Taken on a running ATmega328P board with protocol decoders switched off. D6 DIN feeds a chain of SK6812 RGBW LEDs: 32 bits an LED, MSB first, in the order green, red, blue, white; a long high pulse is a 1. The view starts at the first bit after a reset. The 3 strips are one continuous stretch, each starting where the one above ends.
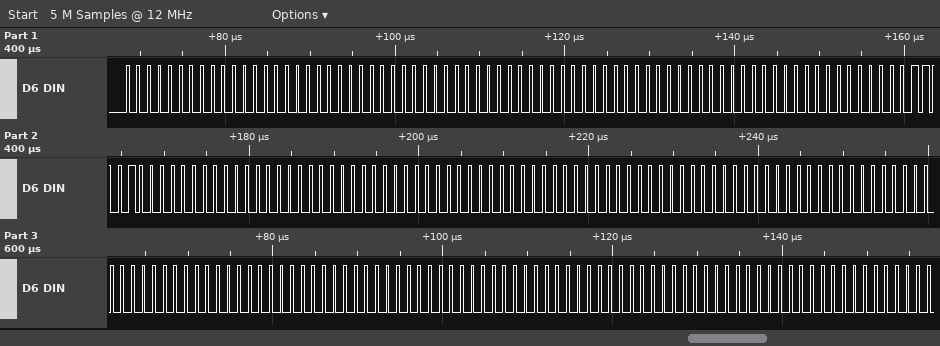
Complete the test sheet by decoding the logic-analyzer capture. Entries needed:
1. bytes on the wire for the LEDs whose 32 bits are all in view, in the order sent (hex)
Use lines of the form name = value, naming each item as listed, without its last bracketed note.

bytes on the wire for the LEDs whose 32 bits are all in view, in the order sent = 00 00 00 00 00 00 00 00 00 32 00 00 00 00 00 00 00 00 00 00 00 00 00 00 00 00 00 00
